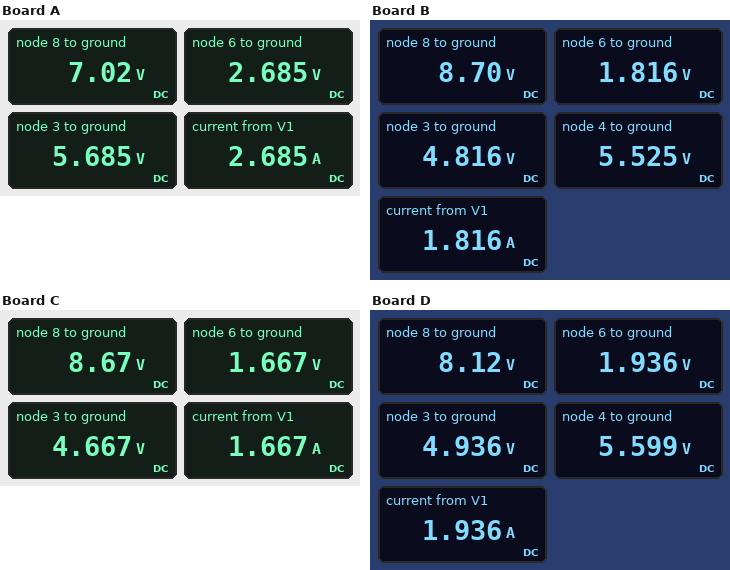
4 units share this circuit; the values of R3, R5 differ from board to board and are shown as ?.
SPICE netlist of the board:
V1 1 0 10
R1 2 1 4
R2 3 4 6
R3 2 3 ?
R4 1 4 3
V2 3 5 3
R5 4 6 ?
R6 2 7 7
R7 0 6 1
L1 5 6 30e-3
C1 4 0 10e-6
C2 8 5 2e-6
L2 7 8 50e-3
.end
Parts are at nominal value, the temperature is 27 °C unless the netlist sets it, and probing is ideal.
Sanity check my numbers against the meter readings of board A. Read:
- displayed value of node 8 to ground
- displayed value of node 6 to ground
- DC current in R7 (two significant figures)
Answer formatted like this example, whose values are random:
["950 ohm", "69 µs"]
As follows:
["7.02 V", "2.685 V", "2.7 A"]
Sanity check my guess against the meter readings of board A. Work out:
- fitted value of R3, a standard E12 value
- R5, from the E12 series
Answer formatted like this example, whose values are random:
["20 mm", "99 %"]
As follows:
["1.8 Ω", "0.68 Ω"]
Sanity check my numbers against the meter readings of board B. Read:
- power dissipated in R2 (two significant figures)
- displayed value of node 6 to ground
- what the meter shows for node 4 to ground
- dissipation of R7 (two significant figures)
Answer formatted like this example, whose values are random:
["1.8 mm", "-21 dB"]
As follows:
["84 mW", "1.816 V", "5.525 V", "3.3 W"]
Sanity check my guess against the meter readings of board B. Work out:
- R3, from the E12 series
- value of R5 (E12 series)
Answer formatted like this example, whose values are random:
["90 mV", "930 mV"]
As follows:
["12 Ω", "2.7 Ω"]
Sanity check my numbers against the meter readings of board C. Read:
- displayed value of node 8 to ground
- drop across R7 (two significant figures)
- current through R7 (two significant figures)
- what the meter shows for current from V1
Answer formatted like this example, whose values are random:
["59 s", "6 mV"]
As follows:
["8.67 V", "1.7 V", "1.7 A", "1.667 A"]
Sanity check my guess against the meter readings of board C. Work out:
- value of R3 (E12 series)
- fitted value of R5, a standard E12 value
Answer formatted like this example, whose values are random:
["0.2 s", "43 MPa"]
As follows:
["12 Ω", "3.9 Ω"]
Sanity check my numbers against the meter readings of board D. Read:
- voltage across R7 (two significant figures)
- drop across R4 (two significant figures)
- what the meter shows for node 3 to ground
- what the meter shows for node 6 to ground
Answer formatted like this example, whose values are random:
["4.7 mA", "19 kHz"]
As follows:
["1.9 V", "4.4 V", "4.936 V", "1.936 V"]
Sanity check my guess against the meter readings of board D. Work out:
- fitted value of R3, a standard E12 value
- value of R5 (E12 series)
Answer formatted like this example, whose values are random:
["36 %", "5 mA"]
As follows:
["6.8 Ω", "2.7 Ω"]
